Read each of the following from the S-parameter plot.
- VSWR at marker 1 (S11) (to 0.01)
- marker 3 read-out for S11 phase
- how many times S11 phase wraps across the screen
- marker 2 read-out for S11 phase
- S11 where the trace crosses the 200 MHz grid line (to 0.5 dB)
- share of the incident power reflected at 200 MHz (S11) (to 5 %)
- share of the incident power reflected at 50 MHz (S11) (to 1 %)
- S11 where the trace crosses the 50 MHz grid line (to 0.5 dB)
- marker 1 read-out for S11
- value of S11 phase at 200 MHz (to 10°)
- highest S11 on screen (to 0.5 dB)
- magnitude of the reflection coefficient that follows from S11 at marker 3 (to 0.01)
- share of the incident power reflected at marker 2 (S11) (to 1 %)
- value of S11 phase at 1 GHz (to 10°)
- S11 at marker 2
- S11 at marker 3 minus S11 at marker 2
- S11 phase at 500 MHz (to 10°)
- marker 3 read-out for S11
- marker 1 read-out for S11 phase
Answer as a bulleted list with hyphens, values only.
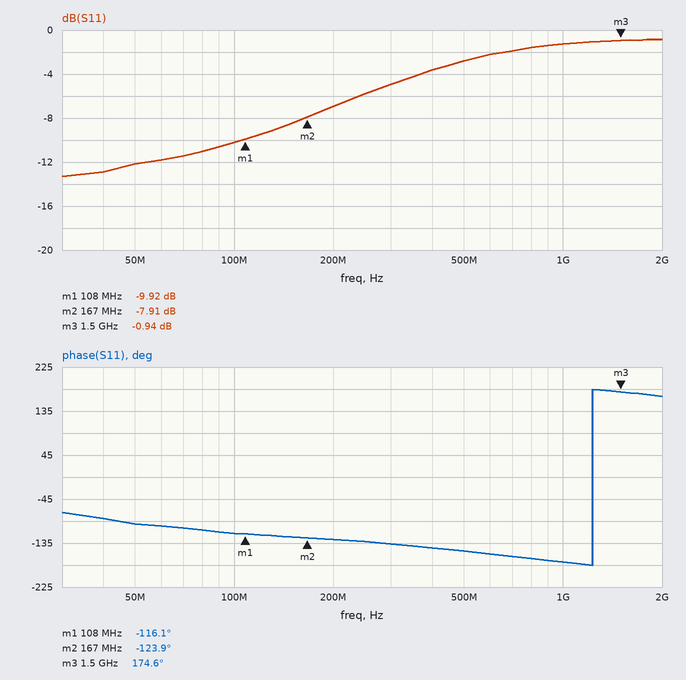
- 1.94
- 174.6°
- 1
- -123.9°
- -7.0 dB
- 20 %
- 6 %
- -12.0 dB
- -9.92 dB
- -130°
- -1.0 dB
- 0.90
- 16 %
- -170°
- -7.91 dB
- 6.97 dB
- -150°
- -0.94 dB
- -116.1°
